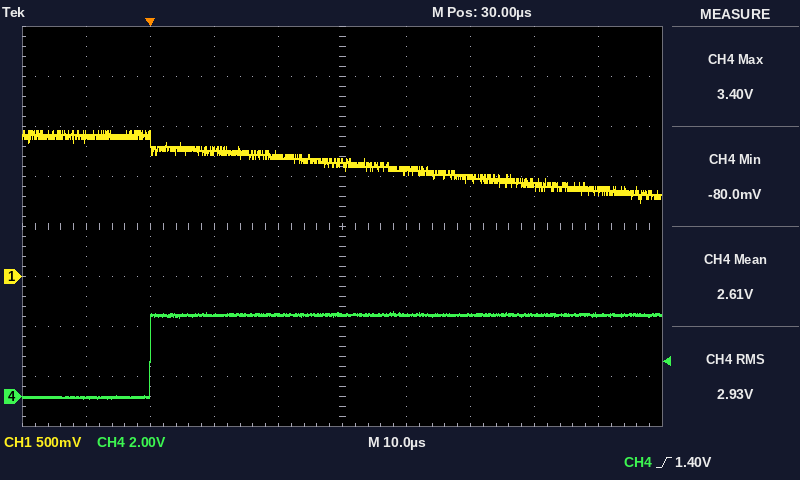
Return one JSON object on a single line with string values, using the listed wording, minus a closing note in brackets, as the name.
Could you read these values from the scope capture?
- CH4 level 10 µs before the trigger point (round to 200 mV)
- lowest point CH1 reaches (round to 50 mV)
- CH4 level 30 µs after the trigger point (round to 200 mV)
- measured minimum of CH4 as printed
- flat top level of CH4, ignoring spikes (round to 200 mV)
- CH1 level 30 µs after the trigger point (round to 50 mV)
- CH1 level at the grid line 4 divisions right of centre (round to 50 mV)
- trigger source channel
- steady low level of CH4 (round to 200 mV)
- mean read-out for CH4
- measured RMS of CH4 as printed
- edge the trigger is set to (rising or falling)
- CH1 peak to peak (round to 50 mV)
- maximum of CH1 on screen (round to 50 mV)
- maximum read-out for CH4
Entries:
{"CH4 level 10 µs before the trigger point": "0.0 V", "lowest point CH1 reaches": "750 mV", "CH4 level 30 µs after the trigger point": "3.2 V", "measured minimum of CH4 as printed": "-80.0 mV", "flat top level of CH4, ignoring spikes": "3.2 V", "CH1 level 30 µs after the trigger point": "1.15 V", "CH1 level at the grid line 4 divisions right of centre": "850 mV", "trigger source channel": "CH4", "steady low level of CH4": "0.0 V", "mean read-out for CH4": "2.61 V", "measured RMS of CH4 as printed": "2.93 V", "edge the trigger is set to": "rising", "CH1 peak to peak": "700 mV", "maximum of CH1 on screen": "1.45 V", "maximum read-out for CH4": "3.40 V"}
